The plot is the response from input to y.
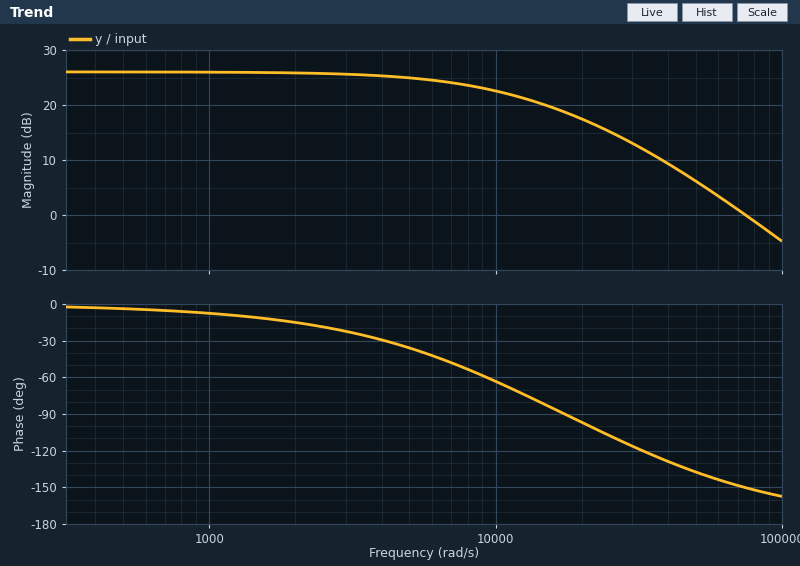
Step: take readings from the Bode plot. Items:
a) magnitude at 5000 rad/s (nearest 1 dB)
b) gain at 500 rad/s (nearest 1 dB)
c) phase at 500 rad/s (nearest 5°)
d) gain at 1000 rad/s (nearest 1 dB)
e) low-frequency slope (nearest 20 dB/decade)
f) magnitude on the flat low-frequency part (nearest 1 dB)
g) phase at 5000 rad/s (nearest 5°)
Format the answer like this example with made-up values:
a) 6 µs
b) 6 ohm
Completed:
a) 25 dB
b) 26 dB
c) -5°
d) 26 dB
e) 0 dB/decade
f) 26 dB
g) -35°
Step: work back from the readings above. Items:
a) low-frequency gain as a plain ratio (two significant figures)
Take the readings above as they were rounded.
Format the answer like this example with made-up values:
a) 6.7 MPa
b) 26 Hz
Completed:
a) 20
